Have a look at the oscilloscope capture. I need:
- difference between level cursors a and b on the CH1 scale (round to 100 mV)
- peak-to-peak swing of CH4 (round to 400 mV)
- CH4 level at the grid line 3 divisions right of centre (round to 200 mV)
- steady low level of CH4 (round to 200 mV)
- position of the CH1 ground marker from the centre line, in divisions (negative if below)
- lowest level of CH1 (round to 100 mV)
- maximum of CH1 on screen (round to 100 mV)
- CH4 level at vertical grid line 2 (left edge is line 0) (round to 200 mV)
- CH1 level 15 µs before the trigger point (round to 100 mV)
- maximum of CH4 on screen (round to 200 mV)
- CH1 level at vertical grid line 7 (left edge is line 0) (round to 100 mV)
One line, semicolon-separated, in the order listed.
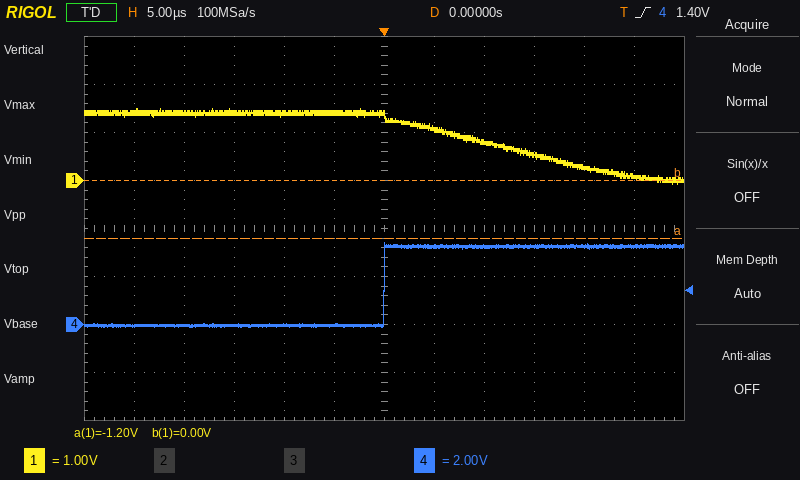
1.2 V; 3.6 V; 3.2 V; 0.0 V; +1.0 div; -100 mV; 1.5 V; 0.0 V; 1.4 V; 3.4 V; 1.1 V
